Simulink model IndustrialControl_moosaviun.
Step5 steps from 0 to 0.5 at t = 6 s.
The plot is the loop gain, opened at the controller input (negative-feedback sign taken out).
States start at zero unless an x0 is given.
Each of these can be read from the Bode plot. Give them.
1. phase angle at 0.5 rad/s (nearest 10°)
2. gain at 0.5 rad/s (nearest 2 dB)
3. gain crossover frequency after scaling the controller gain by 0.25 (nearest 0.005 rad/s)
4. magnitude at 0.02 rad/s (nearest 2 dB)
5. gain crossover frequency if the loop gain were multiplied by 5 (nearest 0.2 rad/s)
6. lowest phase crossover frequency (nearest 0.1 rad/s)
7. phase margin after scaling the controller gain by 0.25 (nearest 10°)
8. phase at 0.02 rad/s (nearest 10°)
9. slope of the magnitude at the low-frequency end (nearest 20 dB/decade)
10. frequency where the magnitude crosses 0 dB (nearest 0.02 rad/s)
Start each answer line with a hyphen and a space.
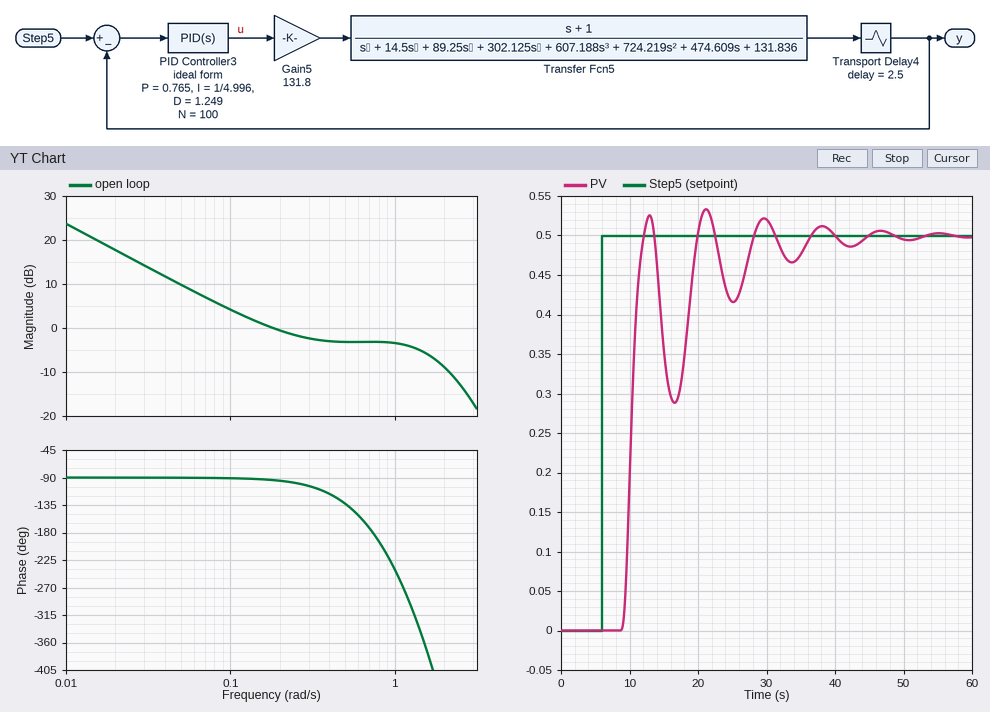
- -130°
- -4 dB
- 0.040 rad/s
- 18 dB
- 2.6 rad/s
- 0.7 rad/s
- 90°
- -90°
- -20 dB/decade
- 0.18 rad/s
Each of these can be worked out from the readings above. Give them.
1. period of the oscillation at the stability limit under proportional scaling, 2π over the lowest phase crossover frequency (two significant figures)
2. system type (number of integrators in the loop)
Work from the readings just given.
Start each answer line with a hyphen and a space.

- 9.0 s
- 1
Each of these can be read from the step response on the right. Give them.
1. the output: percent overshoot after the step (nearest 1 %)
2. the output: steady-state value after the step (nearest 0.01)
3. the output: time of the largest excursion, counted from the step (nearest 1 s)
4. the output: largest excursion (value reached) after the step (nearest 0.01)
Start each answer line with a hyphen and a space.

- 7 %
- 0.50
- 15 s
- 0.53
